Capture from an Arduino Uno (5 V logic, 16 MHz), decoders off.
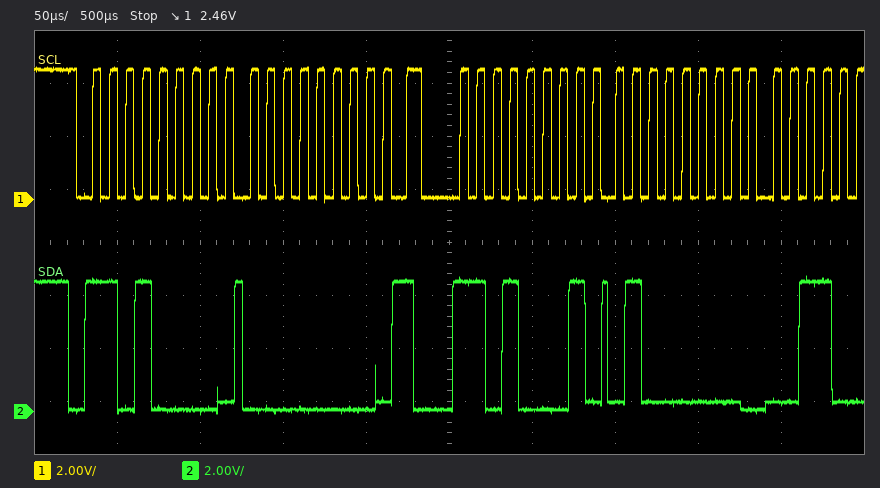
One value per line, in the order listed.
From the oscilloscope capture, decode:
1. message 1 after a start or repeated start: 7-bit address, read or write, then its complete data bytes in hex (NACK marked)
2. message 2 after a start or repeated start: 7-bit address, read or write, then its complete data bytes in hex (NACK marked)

0x68 write: 00
0x68 read: 40
